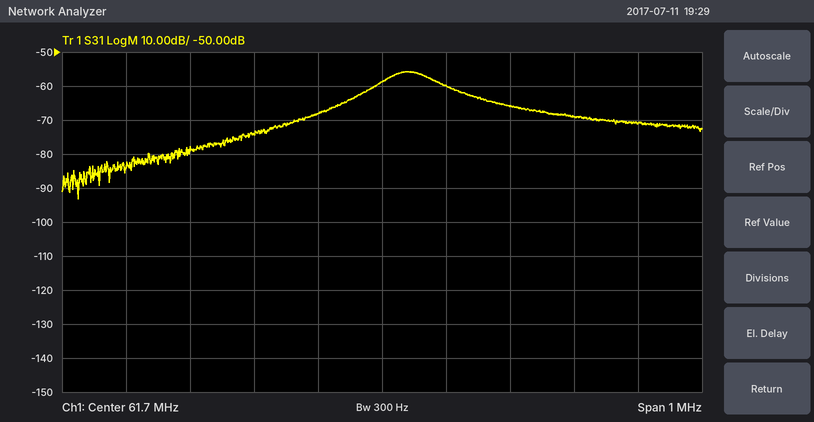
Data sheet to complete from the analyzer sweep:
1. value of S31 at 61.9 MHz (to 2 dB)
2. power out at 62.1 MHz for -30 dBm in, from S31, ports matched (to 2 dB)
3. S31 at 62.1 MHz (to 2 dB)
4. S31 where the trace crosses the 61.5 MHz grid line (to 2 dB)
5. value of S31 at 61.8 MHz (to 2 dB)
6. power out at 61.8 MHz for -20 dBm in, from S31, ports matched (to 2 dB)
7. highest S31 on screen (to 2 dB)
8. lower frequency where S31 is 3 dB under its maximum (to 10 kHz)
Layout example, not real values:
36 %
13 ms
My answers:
-66 dB
-100 dBm
-70 dB
-74 dB
-60 dB
-80 dBm
-56 dB
61.70 MHz
